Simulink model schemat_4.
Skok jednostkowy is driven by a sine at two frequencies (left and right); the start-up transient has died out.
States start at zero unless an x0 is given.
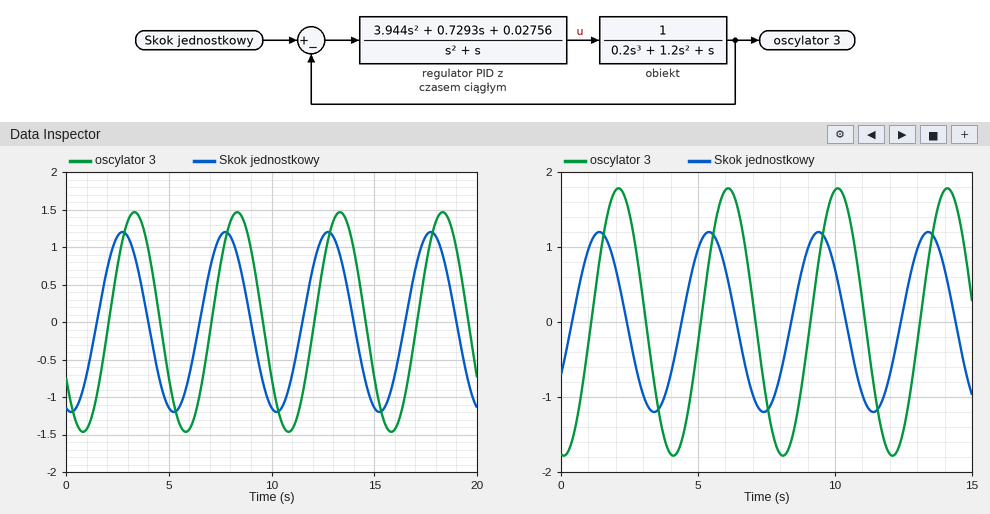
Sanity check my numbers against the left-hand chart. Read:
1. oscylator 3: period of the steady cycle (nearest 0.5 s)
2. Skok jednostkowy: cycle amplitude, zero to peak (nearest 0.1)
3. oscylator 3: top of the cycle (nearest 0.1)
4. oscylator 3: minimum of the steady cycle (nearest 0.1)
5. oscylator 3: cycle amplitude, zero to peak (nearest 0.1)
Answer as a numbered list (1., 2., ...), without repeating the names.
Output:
1. 5.0 s
2. 1.2
3. 1.5
4. -1.5
5. 1.5
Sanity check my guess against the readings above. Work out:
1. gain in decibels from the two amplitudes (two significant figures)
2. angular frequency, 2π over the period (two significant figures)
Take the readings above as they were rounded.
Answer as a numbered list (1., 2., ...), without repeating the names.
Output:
1. 1.9 dB
2. 1.3 rad/s
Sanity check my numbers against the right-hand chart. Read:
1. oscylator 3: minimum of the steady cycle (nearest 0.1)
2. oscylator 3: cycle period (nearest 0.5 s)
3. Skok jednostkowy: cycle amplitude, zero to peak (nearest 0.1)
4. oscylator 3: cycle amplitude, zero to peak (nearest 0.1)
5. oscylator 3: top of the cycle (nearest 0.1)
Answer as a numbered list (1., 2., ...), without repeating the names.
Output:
1. -1.8
2. 4.0 s
3. 1.2
4. 1.8
5. 1.8
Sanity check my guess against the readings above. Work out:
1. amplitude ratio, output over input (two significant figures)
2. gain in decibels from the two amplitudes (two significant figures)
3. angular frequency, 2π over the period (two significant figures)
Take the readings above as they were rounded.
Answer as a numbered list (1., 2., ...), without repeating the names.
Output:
1. 1.5
2. 3.5 dB
3. 1.6 rad/s
